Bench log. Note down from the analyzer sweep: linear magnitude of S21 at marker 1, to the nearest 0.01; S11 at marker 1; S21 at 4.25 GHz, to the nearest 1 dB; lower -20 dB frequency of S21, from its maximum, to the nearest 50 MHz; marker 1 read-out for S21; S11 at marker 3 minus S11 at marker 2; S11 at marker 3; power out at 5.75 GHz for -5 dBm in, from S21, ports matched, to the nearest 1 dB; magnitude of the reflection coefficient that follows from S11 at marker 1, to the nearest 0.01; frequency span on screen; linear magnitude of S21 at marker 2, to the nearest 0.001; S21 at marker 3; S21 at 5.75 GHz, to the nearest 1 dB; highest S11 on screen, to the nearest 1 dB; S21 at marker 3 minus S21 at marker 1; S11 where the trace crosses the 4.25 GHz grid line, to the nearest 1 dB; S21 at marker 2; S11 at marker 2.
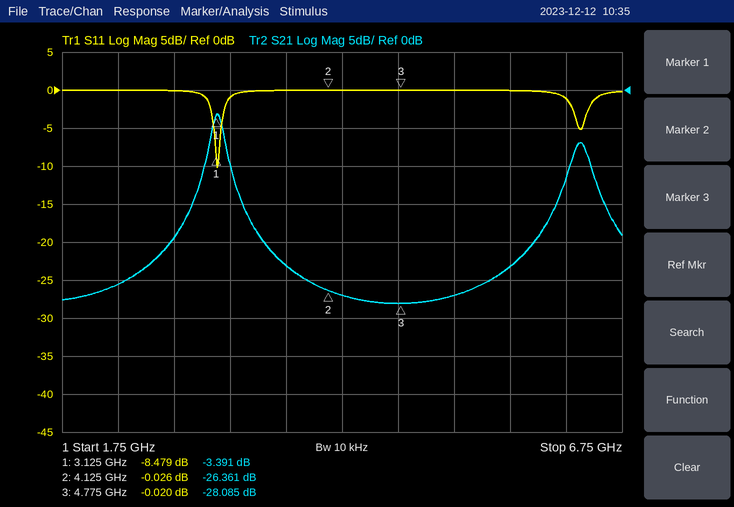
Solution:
0.68
-8.479 dB
-27 dB
2.50 GHz
-3.391 dB
0.006 dB
-0.020 dB
-28 dBm
0.38
5 GHz
0.048
-28.085 dB
-23 dB
0 dB
-24.694 dB
0 dB
-26.361 dB
-0.026 dB
